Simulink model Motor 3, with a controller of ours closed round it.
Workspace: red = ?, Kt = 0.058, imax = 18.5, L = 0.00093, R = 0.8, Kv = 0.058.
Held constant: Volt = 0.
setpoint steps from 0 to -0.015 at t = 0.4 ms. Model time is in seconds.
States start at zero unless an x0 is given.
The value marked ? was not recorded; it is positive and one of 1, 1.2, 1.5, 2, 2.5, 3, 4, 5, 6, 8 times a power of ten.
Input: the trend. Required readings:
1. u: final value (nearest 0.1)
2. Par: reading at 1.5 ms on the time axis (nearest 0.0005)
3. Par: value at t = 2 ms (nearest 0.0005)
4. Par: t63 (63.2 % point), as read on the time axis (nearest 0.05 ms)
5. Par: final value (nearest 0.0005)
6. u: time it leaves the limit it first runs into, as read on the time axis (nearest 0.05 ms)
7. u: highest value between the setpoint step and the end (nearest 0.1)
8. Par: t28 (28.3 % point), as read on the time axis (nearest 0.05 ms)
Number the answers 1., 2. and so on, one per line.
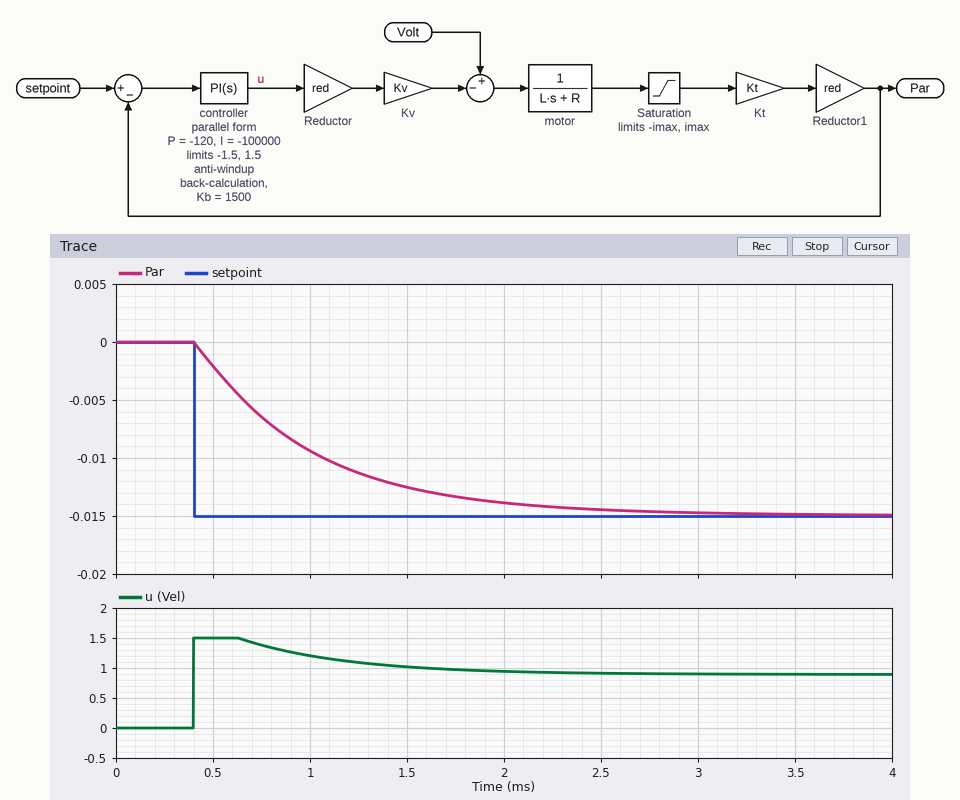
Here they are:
1. 0.9
2. -0.0125
3. -0.0140
4. 1.00 ms
5. -0.0150
6. 0.65 ms
7. 1.5
8. 0.60 ms
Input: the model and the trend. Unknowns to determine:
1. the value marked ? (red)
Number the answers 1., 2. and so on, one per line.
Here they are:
1. 2
